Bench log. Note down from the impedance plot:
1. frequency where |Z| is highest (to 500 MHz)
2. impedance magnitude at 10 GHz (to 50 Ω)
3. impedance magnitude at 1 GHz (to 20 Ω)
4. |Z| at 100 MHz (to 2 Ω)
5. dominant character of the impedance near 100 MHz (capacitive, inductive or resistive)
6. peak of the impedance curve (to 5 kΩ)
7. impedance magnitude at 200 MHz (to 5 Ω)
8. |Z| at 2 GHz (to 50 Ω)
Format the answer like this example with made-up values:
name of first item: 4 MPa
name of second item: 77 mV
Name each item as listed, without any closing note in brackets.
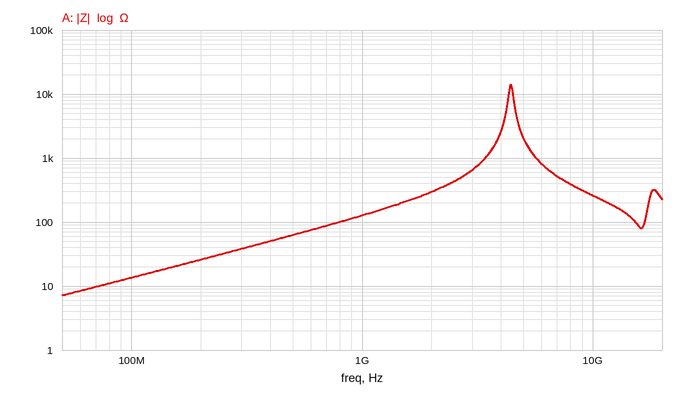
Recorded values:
frequency where |Z| is highest: 4.5 GHz
impedance magnitude at 10 GHz: 250 Ω
impedance magnitude at 1 GHz: 120 Ω
|Z| at 100 MHz: 14 Ω
dominant character of the impedance near 100 MHz: inductive
peak of the impedance curve: 15 kΩ
impedance magnitude at 200 MHz: 25 Ω
|Z| at 2 GHz: 300 Ω
